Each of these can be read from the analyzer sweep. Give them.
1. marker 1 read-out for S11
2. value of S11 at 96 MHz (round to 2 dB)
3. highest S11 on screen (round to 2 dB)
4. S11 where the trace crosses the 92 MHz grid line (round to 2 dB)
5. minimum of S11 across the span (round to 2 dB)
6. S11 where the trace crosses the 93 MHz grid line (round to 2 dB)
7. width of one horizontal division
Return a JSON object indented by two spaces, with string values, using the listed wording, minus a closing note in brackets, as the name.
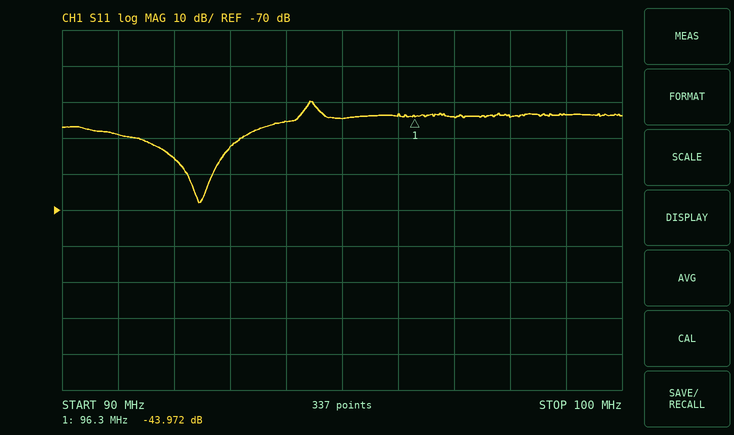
{
  "marker 1 read-out for S11": "-43.972 dB",
  "value of S11 at 96 MHz": "-44 dB",
  "highest S11 on screen": "-40 dB",
  "S11 where the trace crosses the 92 MHz grid line": "-56 dB",
  "minimum of S11 across the span": "-68 dB",
  "S11 where the trace crosses the 93 MHz grid line": "-52 dB",
  "width of one horizontal division": "1 MHz"
}
